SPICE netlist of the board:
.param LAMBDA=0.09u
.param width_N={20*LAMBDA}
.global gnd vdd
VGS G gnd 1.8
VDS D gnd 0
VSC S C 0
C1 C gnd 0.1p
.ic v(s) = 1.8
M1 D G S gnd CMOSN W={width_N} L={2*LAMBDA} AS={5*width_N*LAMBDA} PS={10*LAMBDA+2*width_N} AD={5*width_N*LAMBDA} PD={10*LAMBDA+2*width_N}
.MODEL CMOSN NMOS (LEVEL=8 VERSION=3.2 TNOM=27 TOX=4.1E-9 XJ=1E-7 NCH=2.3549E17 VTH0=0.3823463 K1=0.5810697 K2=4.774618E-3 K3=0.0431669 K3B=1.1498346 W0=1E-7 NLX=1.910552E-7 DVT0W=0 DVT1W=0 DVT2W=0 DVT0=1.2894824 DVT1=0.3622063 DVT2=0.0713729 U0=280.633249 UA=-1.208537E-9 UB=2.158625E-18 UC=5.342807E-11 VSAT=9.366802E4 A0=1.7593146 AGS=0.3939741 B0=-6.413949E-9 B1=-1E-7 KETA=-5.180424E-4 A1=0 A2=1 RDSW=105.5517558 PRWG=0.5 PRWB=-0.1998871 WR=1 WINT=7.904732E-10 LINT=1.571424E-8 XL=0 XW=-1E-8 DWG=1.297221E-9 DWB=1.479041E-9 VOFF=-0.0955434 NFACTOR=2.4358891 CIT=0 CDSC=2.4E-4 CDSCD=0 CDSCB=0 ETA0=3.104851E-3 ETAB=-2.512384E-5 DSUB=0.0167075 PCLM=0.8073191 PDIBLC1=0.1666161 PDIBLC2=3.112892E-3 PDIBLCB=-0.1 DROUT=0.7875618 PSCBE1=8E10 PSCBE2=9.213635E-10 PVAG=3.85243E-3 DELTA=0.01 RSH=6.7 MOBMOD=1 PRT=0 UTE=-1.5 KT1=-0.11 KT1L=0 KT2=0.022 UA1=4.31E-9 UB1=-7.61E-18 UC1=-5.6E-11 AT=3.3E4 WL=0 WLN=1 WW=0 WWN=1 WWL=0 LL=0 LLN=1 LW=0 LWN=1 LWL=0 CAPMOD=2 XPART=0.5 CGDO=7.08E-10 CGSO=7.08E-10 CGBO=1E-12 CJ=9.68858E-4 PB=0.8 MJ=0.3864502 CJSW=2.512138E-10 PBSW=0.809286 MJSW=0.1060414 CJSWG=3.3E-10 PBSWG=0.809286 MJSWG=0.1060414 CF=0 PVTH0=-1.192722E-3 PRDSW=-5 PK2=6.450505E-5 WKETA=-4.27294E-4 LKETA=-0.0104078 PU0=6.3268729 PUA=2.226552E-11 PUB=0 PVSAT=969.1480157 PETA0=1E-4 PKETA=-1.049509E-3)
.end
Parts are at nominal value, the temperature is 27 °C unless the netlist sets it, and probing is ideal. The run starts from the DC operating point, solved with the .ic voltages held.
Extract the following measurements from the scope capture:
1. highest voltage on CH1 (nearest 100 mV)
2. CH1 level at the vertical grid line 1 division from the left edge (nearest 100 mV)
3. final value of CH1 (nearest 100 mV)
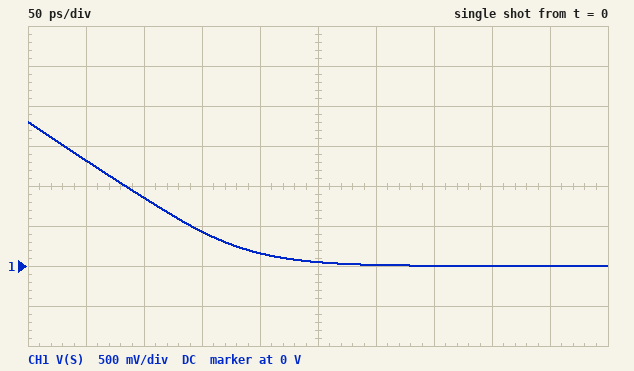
1.8 V
1.3 V
0 V
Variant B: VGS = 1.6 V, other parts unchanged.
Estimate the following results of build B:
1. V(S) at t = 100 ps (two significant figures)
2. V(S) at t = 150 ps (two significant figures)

1.0 V
640 mV
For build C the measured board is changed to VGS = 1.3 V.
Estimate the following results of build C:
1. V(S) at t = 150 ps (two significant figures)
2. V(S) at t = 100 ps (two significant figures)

1.0 V
1.3 V
